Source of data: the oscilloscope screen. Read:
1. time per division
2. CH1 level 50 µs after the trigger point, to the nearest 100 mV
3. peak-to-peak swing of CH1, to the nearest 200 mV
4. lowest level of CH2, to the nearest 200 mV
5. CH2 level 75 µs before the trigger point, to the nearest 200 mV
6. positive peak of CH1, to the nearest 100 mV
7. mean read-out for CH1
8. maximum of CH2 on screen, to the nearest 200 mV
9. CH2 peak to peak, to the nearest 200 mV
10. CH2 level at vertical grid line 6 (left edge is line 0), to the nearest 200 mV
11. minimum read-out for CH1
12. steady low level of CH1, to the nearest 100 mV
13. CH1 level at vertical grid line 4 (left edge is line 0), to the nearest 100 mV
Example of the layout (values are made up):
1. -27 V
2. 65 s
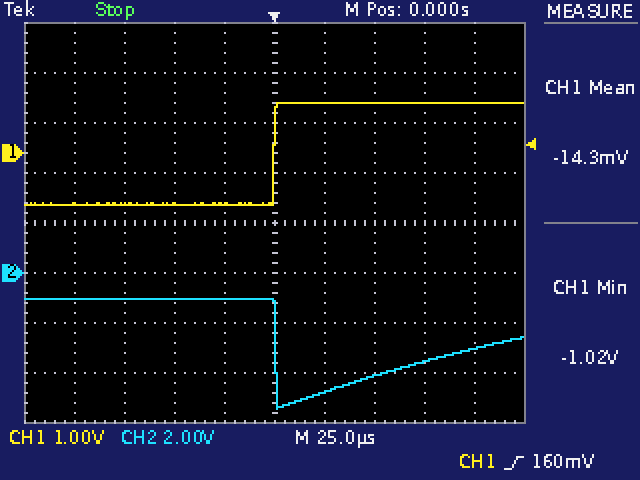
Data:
1. 25 µs
2. 1.0 V
3. 2.0 V
4. -5.4 V
5. -1.0 V
6. 1.0 V
7. -14.3 mV
8. -1.0 V
9. 4.4 V
10. -4.8 V
11. -1.02 V
12. -1.0 V
13. -1.0 V
